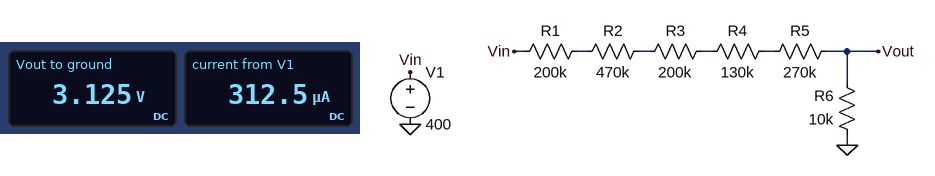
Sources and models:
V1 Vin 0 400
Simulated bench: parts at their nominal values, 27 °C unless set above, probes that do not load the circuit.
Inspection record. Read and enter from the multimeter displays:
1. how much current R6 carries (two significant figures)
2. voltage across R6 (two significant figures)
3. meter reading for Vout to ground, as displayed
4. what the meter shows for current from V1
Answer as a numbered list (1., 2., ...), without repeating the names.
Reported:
1. 310 µA
2. 3.1 V
3. 3.125 V
4. 312.5 µA
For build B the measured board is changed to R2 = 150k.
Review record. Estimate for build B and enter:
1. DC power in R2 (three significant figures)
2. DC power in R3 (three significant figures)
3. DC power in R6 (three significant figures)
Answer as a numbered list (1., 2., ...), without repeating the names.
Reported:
1. 26.0 mW
2. 34.7 mW
3. 1.74 mW
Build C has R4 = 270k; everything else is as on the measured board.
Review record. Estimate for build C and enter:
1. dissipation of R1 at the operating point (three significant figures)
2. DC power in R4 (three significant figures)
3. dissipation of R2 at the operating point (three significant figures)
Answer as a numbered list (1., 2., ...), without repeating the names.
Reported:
1. 15.9 mW
2. 21.4 mW
3. 37.3 mW
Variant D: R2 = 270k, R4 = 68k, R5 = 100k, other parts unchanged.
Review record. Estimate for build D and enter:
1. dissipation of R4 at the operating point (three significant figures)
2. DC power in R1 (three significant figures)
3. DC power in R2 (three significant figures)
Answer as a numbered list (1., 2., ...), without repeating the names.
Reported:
1. 15.1 mW
2. 44.5 mW
3. 60.1 mW
